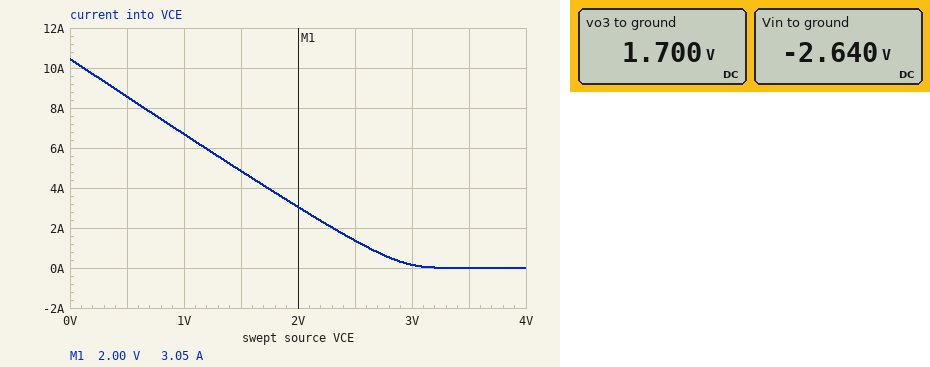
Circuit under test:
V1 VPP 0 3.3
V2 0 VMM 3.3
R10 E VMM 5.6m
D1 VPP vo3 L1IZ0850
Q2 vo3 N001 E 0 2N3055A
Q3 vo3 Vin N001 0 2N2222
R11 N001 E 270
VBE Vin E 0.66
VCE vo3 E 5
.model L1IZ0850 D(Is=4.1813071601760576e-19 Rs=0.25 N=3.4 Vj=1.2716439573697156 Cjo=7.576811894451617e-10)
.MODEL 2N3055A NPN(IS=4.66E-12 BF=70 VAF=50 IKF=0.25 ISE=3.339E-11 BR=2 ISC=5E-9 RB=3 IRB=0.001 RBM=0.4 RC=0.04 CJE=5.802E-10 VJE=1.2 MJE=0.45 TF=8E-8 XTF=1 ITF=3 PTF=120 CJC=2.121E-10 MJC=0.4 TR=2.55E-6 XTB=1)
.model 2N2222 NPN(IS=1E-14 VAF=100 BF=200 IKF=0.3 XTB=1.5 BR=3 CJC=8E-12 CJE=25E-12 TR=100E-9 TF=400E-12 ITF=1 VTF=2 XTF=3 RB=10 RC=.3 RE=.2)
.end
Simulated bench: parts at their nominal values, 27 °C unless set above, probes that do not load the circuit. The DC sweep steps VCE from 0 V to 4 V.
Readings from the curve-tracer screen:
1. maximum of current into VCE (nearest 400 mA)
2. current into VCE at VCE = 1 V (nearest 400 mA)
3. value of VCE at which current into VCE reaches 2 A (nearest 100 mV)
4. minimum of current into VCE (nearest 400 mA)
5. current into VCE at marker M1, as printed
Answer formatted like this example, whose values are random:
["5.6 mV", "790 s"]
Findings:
["10.4 A", "6.8 A", "2.3 V", "0 A", "3.05 A"]
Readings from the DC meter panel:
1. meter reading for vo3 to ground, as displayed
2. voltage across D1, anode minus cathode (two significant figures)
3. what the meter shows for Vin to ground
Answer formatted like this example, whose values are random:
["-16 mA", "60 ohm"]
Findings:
["1.700 V", "1.6 V", "-2.640 V"]
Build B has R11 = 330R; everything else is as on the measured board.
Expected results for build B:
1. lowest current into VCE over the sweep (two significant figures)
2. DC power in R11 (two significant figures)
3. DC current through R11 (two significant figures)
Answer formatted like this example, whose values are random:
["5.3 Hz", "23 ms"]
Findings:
["-160 µA", "8.6 µW", "160 µA"]
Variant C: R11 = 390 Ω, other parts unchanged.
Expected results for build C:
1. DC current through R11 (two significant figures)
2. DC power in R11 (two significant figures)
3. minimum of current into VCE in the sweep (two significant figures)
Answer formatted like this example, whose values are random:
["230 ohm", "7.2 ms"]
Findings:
["140 µA", "8.1 µW", "-140 µA"]
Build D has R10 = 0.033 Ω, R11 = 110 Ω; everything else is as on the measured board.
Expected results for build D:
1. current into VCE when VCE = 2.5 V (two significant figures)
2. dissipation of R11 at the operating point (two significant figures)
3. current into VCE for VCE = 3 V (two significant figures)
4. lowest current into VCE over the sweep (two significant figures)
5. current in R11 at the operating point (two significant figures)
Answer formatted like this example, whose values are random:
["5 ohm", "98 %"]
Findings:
["1.3 A", "11 µW", "150 mA", "-320 µA", "320 µA"]
